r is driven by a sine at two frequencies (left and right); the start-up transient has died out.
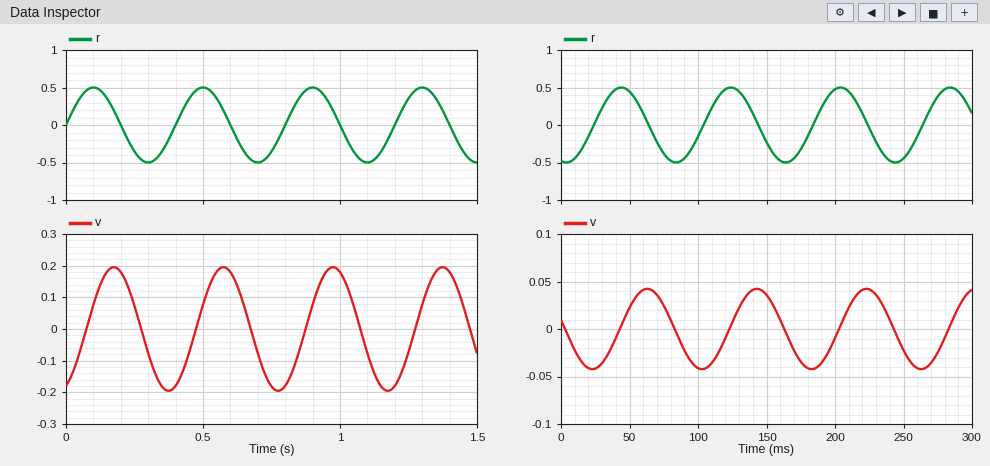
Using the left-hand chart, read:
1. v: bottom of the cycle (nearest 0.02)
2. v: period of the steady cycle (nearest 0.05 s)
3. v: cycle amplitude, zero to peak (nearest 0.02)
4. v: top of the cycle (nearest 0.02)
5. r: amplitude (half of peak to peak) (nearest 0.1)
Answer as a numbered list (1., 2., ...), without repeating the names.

1. -0.20
2. 0.40 s
3. 0.20
4. 0.20
5. 0.5
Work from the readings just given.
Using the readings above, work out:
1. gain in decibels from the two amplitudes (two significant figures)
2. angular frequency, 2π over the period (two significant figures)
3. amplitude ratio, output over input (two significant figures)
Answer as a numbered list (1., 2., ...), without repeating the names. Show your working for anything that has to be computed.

1. 20 log10(0.2 / 0.5) = -8.0 dB
2. 2π / 0.4 = 16 rad/s
3. 0.2 / 0.5 = 0.40
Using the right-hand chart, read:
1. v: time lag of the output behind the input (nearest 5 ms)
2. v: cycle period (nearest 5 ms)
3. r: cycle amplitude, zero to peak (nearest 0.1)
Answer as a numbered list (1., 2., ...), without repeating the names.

1. 20 ms
2. 80 ms
3. 0.5
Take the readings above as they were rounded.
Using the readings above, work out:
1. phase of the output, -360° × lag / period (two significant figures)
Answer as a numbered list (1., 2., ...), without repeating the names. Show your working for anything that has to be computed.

1. -360 × 20 / 80 = -90°
